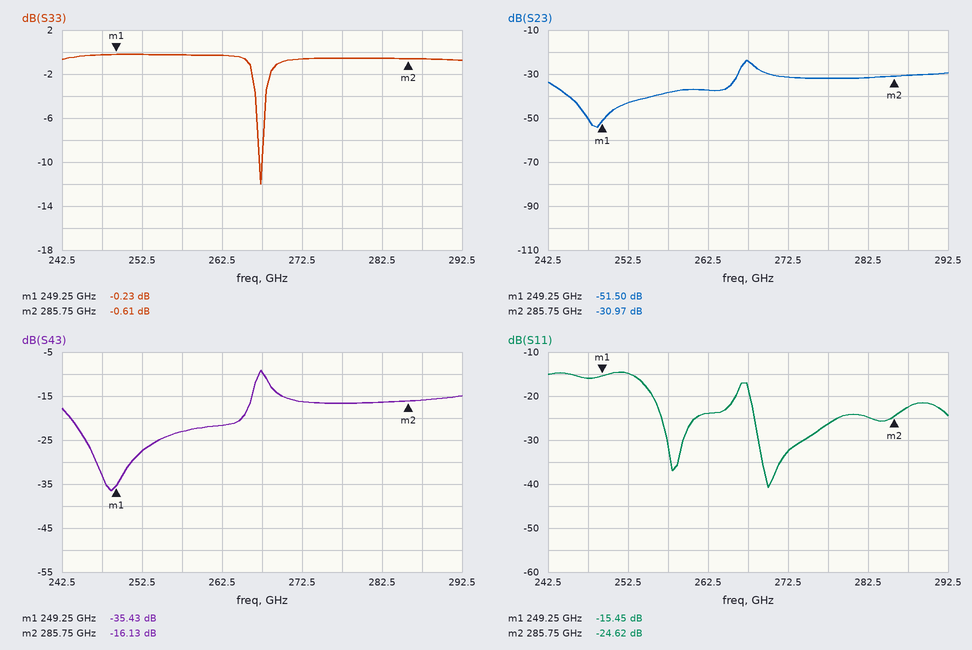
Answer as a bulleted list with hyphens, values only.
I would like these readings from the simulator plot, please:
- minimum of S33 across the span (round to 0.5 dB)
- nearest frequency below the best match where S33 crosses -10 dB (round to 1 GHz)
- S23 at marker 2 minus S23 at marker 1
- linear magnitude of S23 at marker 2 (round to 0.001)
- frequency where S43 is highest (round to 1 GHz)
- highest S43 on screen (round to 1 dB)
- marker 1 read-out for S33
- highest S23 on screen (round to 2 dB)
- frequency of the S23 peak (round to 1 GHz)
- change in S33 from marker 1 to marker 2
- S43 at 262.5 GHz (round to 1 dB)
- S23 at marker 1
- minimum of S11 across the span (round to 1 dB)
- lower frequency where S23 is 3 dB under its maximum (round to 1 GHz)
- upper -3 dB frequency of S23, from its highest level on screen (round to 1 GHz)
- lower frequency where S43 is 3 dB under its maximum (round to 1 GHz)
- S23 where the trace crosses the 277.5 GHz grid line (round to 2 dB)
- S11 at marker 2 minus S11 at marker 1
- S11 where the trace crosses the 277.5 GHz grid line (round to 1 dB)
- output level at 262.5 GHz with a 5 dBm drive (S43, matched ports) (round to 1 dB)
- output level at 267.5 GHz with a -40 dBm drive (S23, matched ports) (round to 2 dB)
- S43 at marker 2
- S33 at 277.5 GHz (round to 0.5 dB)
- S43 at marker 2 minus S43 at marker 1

- -12.0 dB
- 267 GHz
- 20.53 dB
- 0.028
- 267 GHz
- -9 dB
- -0.23 dB
- -24 dB
- 267 GHz
- -0.38 dB
- -22 dB
- -51.50 dB
- -41 dB
- 267 GHz
- 268 GHz
- 267 GHz
- -32 dB
- -9.17 dB
- -26 dB
- -17 dBm
- -64 dBm
- -16.13 dB
- -0.5 dB
- 19.30 dB
